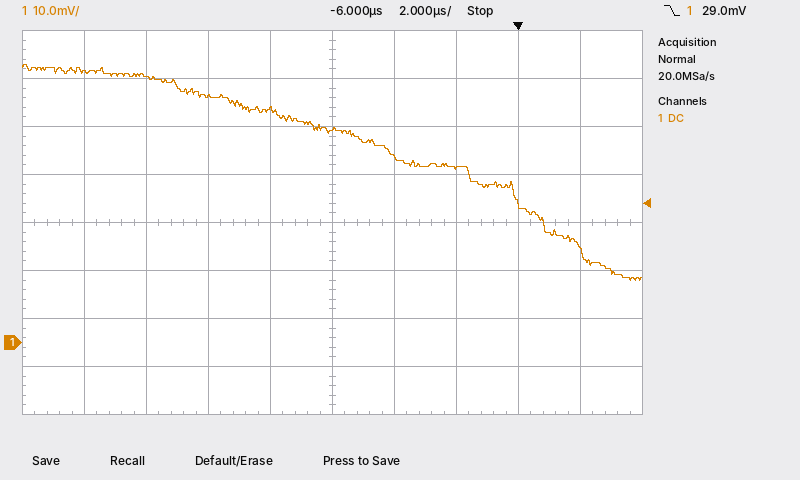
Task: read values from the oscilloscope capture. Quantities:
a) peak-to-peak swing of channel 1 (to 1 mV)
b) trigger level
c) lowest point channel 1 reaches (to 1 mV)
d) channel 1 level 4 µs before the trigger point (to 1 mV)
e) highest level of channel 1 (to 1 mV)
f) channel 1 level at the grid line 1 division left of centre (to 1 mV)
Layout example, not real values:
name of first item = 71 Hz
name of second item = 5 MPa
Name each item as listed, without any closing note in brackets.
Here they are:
peak-to-peak swing of channel 1 = 45 mV
trigger level = 29.0 mV
lowest point channel 1 reaches = 13 mV
channel 1 level 4 µs before the trigger point = 39 mV
highest level of channel 1 = 58 mV
channel 1 level at the grid line 1 division left of centre = 49 mV
